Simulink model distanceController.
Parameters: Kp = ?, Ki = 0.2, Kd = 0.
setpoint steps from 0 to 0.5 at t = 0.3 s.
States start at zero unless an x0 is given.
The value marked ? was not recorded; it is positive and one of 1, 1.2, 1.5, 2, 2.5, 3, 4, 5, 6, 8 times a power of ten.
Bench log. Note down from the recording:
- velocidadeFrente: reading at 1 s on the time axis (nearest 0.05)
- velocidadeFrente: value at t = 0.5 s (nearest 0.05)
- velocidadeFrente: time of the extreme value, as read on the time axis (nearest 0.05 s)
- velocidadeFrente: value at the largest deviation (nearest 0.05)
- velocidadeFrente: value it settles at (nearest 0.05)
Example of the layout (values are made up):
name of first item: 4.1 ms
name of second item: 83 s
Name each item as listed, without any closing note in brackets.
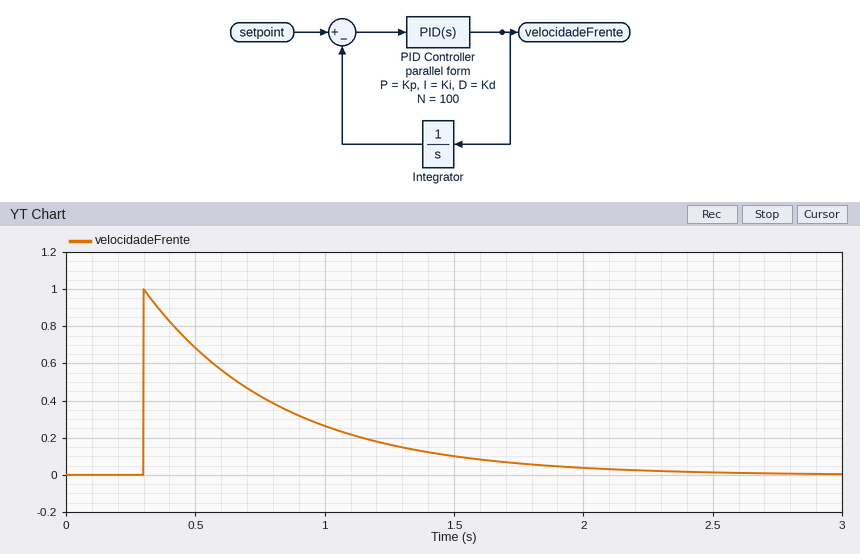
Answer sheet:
velocidadeFrente: reading at 1 s on the time axis: 0.25
velocidadeFrente: value at t = 0.5 s: 0.70
velocidadeFrente: time of the extreme value, as read on the time axis: 0.30 s
velocidadeFrente: value at the largest deviation: 1.00
velocidadeFrente: value it settles at: 0.00
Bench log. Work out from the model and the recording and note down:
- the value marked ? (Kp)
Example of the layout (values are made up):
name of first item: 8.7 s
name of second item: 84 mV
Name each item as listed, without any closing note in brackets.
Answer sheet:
the value marked ?: 2
